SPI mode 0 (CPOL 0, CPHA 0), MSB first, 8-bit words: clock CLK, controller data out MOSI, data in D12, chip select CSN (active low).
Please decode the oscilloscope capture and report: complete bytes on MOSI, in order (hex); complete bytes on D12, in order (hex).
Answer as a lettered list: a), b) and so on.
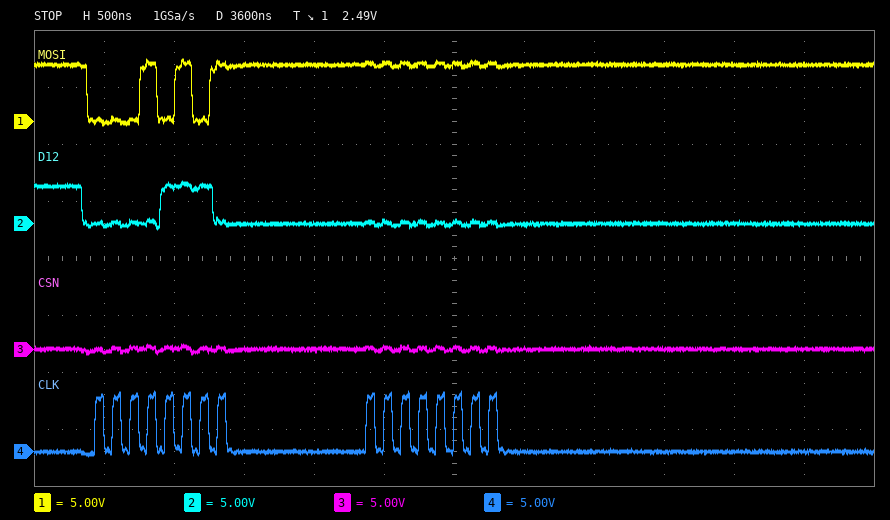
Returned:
a) 15 FF
b) 0E 00
